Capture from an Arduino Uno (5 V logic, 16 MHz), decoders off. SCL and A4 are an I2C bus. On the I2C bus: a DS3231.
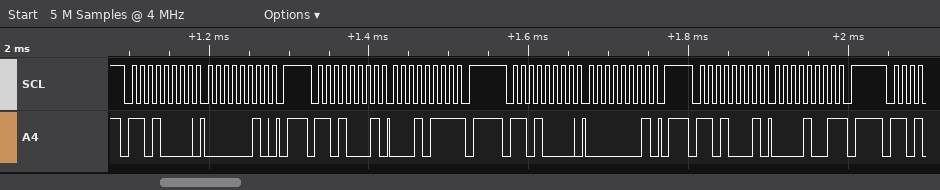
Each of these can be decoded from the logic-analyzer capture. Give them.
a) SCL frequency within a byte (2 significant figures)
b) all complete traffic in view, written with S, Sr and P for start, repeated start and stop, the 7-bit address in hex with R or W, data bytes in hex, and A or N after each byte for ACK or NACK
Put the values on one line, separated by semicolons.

100 kHz; S 68W A 02 A P S 68R A 17 N P S 68W A 01 A P S 68R A 09 N P
